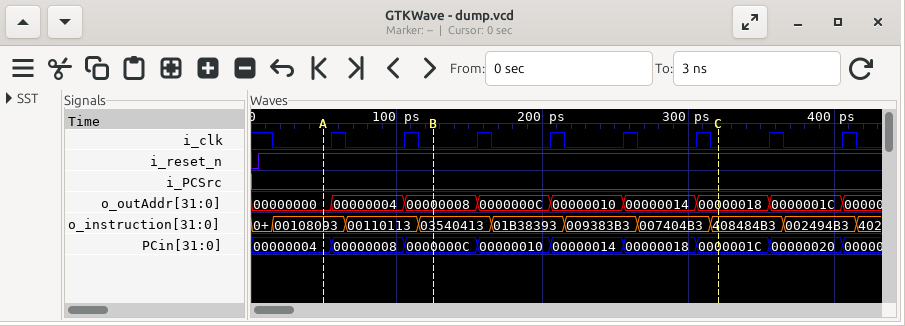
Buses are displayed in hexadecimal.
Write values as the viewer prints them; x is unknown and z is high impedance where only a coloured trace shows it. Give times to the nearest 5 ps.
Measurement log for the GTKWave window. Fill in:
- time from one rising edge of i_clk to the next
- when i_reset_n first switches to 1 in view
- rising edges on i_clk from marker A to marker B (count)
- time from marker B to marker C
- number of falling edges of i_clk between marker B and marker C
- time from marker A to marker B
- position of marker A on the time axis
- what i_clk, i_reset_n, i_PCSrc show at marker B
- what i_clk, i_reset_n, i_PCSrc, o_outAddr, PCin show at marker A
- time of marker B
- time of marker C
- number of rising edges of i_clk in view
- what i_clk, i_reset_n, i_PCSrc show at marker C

50 ps
5 ps
2
195 ps
4
75 ps
50 ps
i_clk=0, i_reset_n=1, i_PCSrc=0
i_clk=0, i_reset_n=1, i_PCSrc=0, o_outAddr=00000000, PCin=00000004
125 ps
320 ps
8
i_clk=0, i_reset_n=1, i_PCSrc=0
